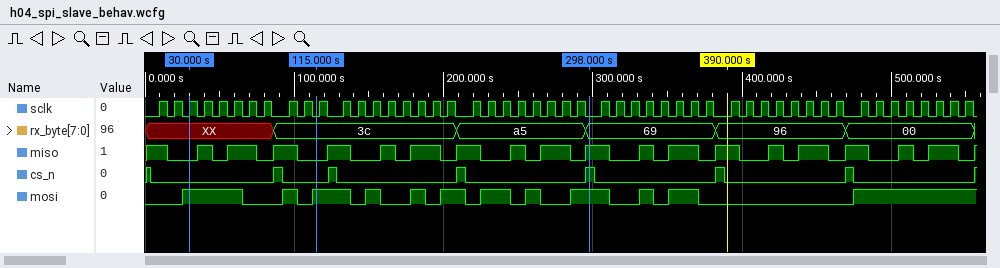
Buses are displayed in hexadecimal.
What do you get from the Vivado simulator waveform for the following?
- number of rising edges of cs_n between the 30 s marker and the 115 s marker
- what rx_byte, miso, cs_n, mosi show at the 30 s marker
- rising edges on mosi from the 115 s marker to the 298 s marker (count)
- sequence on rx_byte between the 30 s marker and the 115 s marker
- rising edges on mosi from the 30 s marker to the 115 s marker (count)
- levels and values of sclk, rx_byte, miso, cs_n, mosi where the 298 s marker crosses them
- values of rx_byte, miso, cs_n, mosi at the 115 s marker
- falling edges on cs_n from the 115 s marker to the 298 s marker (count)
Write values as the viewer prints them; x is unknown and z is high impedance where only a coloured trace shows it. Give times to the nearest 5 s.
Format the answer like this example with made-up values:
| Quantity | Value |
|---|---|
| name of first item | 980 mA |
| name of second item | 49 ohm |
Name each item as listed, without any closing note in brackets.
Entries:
| Quantity | Value |
|---|---|
| number of rising edges of cs_n between the 30 s marker and the 115 s marker | 1 |
| what rx_byte, miso, cs_n, mosi show at the 30 s marker | rx_byte=XX, miso=0, cs_n=0, mosi=1 |
| rising edges on mosi from the 115 s marker to the 298 s marker | 6 |
| sequence on rx_byte between the 30 s marker and the 115 s marker | XX, 3c |
| rising edges on mosi from the 30 s marker to the 115 s marker | 2 |
| levels and values of sclk, rx_byte, miso, cs_n, mosi where the 298 s marker crosses them | sclk=0, rx_byte=69, miso=1, cs_n=1, mosi=1 |
| values of rx_byte, miso, cs_n, mosi at the 115 s marker | rx_byte=3c, miso=0, cs_n=0, mosi=1 |
| falling edges on cs_n from the 115 s marker to the 298 s marker | 2 |
